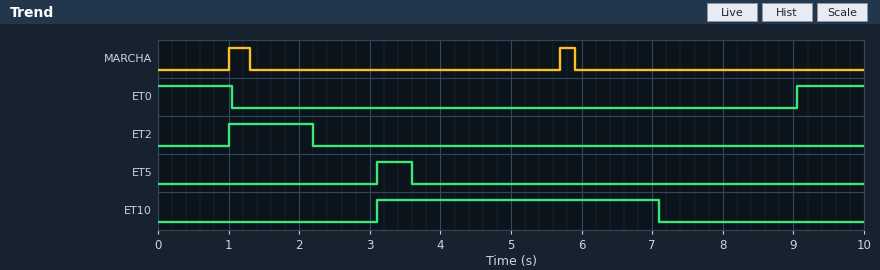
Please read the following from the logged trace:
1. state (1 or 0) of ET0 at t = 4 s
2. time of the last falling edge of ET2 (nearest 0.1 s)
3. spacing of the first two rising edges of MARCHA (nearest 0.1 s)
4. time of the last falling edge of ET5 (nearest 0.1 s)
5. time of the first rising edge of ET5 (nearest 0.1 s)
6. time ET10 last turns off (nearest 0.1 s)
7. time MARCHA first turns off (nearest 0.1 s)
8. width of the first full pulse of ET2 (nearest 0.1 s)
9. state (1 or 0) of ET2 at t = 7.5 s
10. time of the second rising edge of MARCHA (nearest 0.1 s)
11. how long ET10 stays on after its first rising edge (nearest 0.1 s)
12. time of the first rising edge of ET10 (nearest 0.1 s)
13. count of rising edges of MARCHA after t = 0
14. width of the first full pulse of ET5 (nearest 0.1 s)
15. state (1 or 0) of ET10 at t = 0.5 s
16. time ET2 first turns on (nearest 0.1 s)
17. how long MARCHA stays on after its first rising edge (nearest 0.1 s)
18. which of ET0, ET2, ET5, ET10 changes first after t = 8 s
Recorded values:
0
2.2 s
4.7 s
3.6 s
3.1 s
7.1 s
1.3 s
1.2 s
0
5.7 s
4.0 s
3.1 s
2
0.5 s
0
1.0 s
0.3 s
ET0
